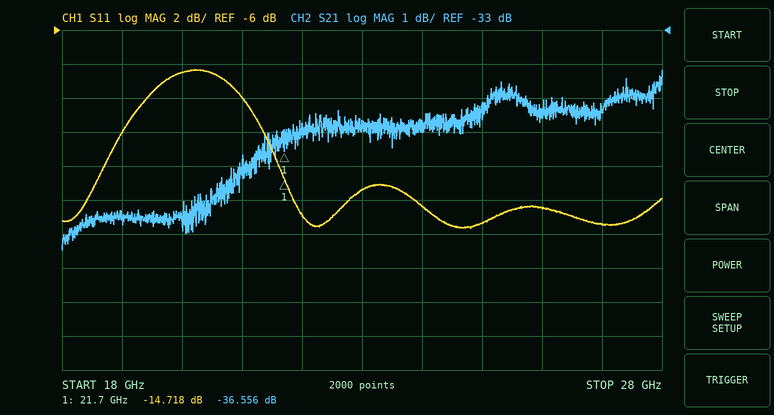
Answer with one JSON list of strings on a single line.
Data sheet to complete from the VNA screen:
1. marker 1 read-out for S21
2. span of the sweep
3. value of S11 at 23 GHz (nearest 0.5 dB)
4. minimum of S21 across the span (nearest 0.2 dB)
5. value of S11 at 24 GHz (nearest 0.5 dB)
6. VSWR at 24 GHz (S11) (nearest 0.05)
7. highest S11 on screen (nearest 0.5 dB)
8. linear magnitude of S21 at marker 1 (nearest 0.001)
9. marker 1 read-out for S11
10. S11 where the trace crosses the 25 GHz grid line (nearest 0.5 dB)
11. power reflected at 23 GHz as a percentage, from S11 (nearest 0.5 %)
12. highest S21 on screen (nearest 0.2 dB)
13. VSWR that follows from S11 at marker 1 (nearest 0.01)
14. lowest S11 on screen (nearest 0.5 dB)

["-36.556 dB", "10 GHz", "-15.5 dB", "-39.4 dB", "-16.5 dB", "1.35", "-8.5 dB", "0.015", "-14.718 dB", "-17.5 dB", "3.0 %", "-34.2 dB", "1.45", "-17.5 dB"]
